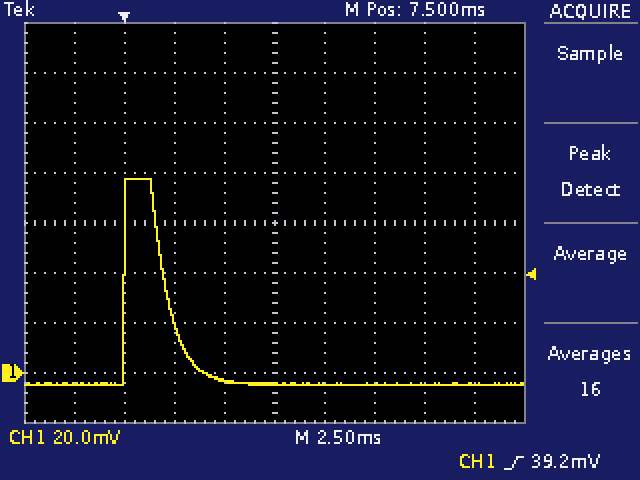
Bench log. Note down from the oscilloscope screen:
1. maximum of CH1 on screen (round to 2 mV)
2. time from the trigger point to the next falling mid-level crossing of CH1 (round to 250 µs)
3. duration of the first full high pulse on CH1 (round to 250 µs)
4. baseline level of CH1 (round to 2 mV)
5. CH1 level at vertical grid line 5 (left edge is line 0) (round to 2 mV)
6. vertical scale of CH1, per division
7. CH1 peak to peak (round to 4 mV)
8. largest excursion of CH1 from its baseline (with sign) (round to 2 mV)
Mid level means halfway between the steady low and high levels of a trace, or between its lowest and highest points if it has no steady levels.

78 mV
2.00 ms
2.00 ms
-4 mV
-4 mV
20 mV
84 mV
+82 mV
